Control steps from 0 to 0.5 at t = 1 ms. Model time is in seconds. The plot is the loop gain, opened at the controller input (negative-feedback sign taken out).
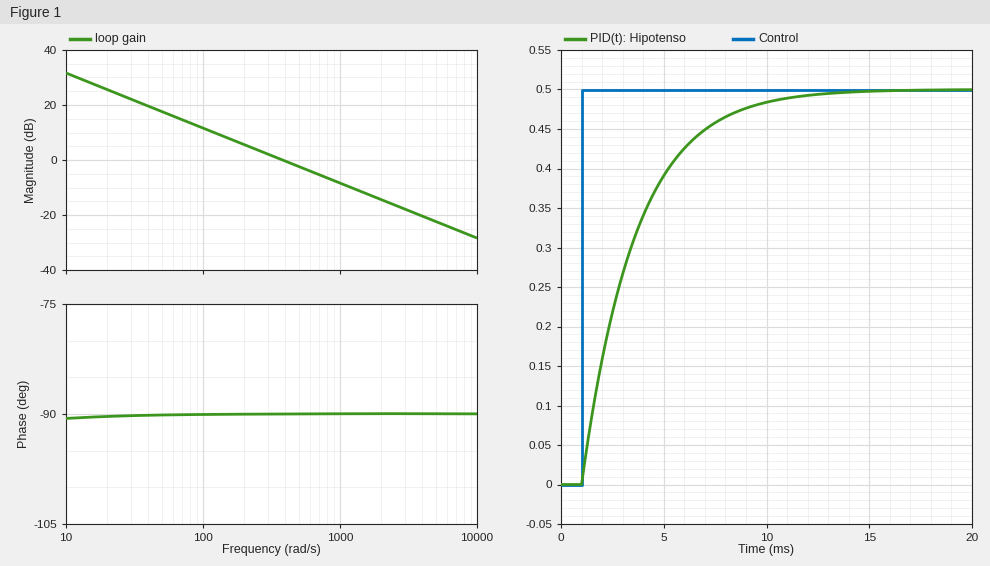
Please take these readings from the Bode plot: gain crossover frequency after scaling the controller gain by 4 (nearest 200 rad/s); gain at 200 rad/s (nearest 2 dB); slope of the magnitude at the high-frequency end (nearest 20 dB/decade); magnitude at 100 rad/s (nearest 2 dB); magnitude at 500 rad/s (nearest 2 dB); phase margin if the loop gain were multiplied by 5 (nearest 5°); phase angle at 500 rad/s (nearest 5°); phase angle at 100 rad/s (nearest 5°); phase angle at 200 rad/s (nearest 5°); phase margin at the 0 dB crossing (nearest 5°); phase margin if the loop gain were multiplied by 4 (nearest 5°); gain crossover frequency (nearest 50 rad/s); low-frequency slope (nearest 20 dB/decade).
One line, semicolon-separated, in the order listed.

1600 rad/s; 6 dB; -20 dB/decade; 12 dB; -2 dB; 90°; -90°; -90°; -90°; 90°; 90°; 400 rad/s; -20 dB/decade
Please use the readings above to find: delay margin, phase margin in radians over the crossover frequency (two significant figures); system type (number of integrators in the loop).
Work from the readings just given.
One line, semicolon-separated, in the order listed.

0.0039 s; 1
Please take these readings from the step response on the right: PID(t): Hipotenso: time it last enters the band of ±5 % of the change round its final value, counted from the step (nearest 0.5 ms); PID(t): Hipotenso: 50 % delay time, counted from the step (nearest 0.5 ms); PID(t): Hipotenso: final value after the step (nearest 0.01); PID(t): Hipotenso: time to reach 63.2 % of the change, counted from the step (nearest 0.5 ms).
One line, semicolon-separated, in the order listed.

8.0 ms; 2.0 ms; 0.50; 2.5 ms
